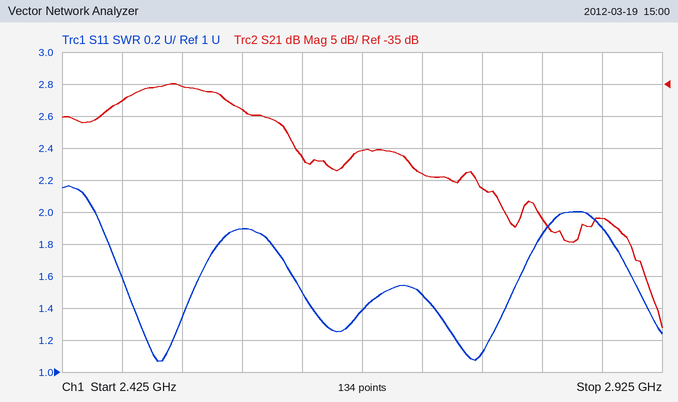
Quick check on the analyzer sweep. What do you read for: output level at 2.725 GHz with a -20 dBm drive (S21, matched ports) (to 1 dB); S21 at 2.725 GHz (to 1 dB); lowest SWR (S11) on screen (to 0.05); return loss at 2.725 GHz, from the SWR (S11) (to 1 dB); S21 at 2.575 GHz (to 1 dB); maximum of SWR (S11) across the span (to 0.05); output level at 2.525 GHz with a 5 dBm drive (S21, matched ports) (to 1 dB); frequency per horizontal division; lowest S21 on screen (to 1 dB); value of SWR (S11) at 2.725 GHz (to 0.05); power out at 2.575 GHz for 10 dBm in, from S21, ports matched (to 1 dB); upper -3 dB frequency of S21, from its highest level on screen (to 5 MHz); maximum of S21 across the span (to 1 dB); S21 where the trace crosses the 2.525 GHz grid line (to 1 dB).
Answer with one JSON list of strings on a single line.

["-69 dBm", "-49 dB", "1.05", "14 dB", "-39 dB", "2.15", "-30 dBm", "50 MHz", "-73 dB", "1.50", "-29 dBm", "2.565 GHz", "-35 dB", "-35 dB"]
